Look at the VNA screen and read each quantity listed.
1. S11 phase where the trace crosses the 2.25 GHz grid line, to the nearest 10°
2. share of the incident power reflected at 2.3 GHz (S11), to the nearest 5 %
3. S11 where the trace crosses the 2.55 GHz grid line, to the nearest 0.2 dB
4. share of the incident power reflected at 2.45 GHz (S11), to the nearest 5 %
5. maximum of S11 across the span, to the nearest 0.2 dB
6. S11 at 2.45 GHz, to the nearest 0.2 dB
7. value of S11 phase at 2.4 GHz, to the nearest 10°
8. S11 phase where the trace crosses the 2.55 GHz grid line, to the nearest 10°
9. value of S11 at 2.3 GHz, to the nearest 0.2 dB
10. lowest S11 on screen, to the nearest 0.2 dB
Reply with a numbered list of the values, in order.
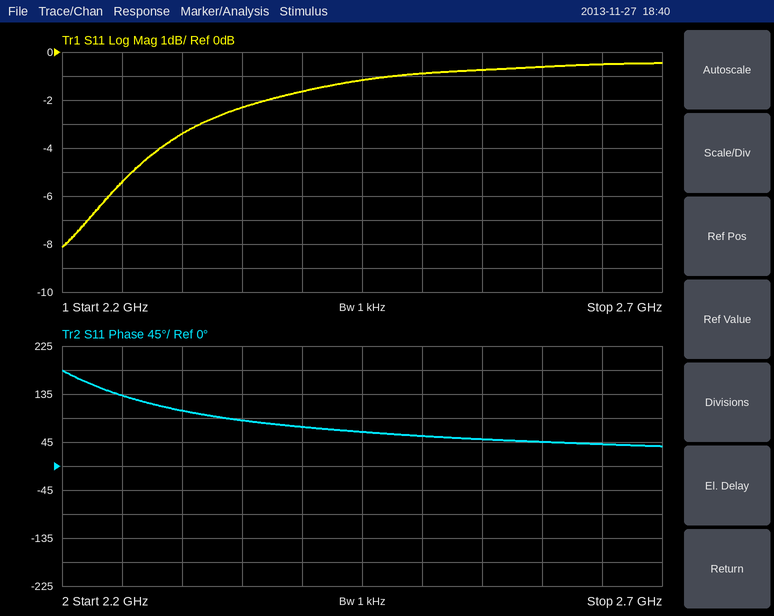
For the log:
1. 130°
2. 45 %
3. -0.8 dB
4. 75 %
5. -0.4 dB
6. -1.2 dB
7. 70°
8. 50°
9. -3.4 dB
10. -8.2 dB
